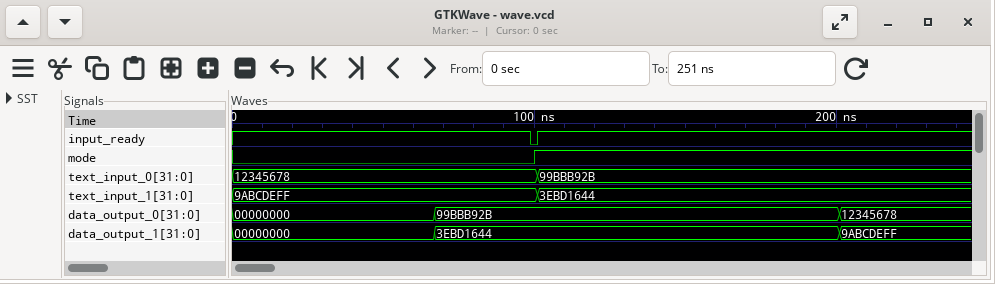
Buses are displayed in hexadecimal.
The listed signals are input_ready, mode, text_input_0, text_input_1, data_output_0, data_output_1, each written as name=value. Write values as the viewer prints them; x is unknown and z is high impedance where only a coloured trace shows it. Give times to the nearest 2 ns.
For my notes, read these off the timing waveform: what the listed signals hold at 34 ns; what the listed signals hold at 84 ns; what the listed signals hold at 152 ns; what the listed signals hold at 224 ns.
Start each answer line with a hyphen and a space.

- input_ready=1, mode=0, text_input_0=12345678, text_input_1=9ABCDEFF, data_output_0=00000000, data_output_1=00000000
- input_ready=1, mode=0, text_input_0=12345678, text_input_1=9ABCDEFF, data_output_0=99BBB92B, data_output_1=3EBD1644
- input_ready=1, mode=1, text_input_0=99BBB92B, text_input_1=3EBD1644, data_output_0=99BBB92B, data_output_1=3EBD1644
- input_ready=1, mode=1, text_input_0=99BBB92B, text_input_1=3EBD1644, data_output_0=12345678, data_output_1=9ABCDEFF
